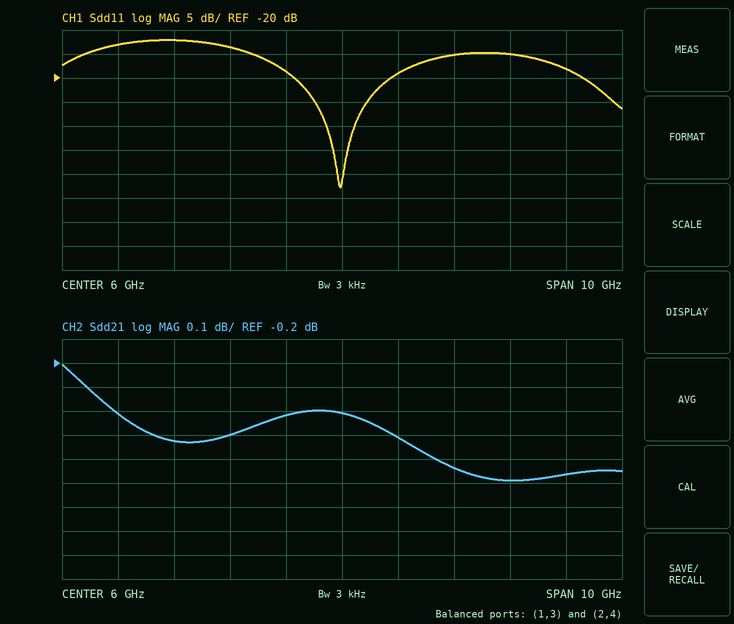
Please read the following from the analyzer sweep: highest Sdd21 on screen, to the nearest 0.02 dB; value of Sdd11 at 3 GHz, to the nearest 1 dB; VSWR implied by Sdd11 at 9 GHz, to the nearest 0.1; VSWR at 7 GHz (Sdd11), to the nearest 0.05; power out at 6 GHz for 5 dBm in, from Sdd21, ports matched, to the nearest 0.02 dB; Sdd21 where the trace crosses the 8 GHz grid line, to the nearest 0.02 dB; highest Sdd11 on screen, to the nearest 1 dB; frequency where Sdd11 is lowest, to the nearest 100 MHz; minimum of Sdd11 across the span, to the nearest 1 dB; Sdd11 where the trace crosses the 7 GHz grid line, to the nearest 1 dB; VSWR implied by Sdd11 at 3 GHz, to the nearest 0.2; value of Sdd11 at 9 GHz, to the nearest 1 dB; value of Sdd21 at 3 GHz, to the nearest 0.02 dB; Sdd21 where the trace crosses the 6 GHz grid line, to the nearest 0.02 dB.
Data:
-0.20 dB
-12 dB
1.4
1.25
4.60 dBm
-0.64 dB
-12 dB
6.0 GHz
-43 dB
-19 dB
1.6
-15 dB
-0.52 dB
-0.40 dB
